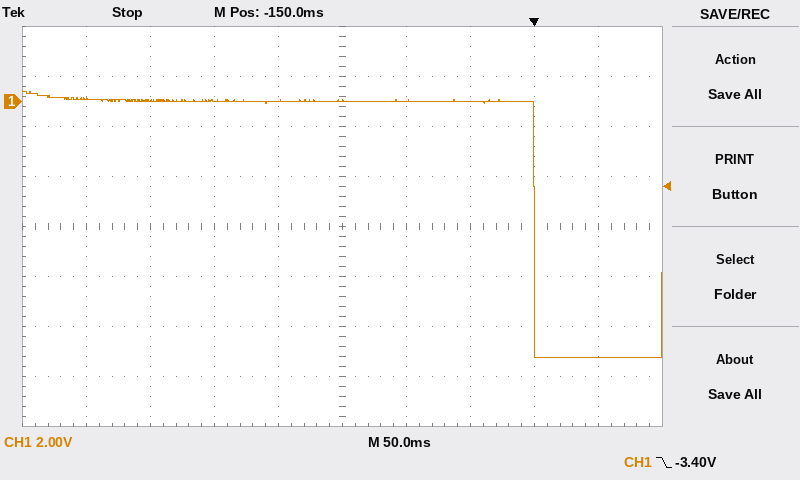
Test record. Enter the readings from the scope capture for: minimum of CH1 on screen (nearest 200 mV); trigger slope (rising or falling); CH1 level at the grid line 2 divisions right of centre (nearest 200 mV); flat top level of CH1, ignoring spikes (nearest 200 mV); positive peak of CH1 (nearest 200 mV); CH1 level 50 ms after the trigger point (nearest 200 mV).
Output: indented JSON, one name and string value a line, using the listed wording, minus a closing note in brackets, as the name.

{
  "minimum of CH1 on screen": "-10.2 V",
  "trigger slope": "falling",
  "CH1 level at the grid line 2 divisions right of centre": "0.0 V",
  "flat top level of CH1, ignoring spikes": "0.0 V",
  "positive peak of CH1": "400 mV",
  "CH1 level 50 ms after the trigger point": "-10.2 V"
}
